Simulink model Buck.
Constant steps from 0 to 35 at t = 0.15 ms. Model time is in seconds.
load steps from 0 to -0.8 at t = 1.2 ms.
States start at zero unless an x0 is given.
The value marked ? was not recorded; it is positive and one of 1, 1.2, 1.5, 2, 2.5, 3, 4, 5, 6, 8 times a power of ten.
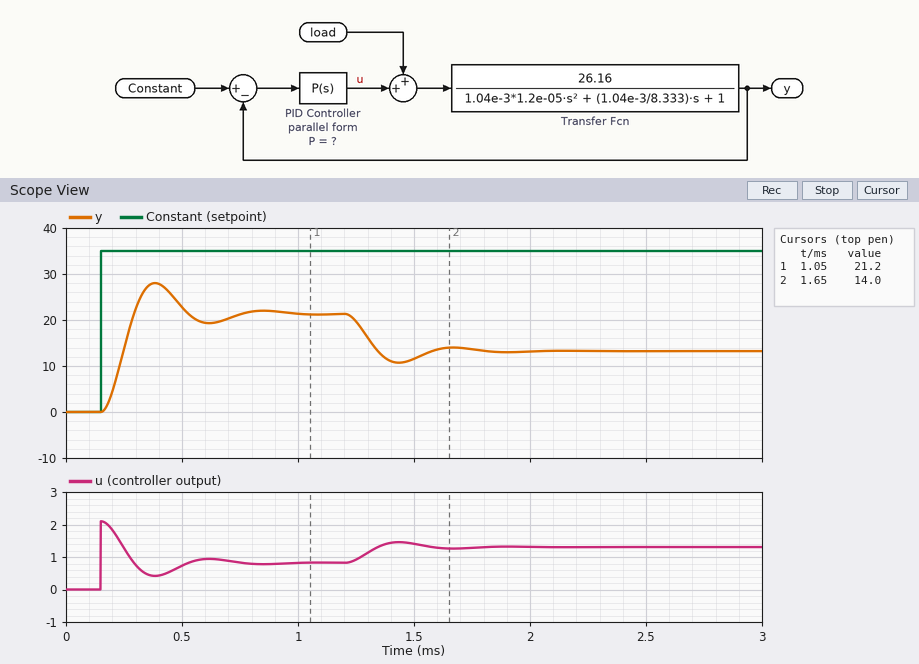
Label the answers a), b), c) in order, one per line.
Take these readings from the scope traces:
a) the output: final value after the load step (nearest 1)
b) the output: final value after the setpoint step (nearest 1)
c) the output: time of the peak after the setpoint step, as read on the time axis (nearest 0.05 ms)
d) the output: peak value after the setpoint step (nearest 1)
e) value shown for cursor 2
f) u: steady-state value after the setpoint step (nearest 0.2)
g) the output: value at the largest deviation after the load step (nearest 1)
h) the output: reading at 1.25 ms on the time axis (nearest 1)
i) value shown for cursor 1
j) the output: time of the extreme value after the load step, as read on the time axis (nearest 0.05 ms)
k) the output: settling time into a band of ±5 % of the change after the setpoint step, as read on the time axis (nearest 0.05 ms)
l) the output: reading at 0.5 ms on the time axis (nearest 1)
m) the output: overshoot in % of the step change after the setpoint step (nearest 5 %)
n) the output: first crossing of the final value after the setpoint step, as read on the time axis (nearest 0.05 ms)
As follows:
a) 13
b) 21
c) 0.40 ms
d) 28
e) 14.0
f) 0.8
g) 11
h) 20
i) 21.2
j) 1.45 ms
k) 0.70 ms
l) 23
m) 30 %
n) 0.30 ms
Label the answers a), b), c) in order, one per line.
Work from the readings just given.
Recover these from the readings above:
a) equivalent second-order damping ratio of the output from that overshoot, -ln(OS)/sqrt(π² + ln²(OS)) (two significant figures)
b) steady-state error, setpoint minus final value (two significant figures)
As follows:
a) 0.36
b) 14
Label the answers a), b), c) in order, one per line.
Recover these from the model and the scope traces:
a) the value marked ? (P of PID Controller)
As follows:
a) 0.06
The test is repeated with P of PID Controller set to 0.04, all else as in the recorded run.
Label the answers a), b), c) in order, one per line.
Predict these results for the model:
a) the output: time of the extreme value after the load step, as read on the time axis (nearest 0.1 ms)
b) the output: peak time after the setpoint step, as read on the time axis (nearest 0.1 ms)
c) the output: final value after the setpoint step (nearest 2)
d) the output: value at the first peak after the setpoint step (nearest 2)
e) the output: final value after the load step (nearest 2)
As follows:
a) 1.5 ms
b) 0.4 ms
c) 18
d) 22
e) 8
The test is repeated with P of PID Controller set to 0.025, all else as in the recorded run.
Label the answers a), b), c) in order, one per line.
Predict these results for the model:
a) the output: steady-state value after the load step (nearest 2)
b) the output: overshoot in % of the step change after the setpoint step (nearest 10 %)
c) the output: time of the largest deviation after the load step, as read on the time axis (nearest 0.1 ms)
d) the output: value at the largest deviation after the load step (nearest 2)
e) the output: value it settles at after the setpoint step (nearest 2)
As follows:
a) 2
b) 20 %
c) 1.5 ms
d) -2
e) 14
